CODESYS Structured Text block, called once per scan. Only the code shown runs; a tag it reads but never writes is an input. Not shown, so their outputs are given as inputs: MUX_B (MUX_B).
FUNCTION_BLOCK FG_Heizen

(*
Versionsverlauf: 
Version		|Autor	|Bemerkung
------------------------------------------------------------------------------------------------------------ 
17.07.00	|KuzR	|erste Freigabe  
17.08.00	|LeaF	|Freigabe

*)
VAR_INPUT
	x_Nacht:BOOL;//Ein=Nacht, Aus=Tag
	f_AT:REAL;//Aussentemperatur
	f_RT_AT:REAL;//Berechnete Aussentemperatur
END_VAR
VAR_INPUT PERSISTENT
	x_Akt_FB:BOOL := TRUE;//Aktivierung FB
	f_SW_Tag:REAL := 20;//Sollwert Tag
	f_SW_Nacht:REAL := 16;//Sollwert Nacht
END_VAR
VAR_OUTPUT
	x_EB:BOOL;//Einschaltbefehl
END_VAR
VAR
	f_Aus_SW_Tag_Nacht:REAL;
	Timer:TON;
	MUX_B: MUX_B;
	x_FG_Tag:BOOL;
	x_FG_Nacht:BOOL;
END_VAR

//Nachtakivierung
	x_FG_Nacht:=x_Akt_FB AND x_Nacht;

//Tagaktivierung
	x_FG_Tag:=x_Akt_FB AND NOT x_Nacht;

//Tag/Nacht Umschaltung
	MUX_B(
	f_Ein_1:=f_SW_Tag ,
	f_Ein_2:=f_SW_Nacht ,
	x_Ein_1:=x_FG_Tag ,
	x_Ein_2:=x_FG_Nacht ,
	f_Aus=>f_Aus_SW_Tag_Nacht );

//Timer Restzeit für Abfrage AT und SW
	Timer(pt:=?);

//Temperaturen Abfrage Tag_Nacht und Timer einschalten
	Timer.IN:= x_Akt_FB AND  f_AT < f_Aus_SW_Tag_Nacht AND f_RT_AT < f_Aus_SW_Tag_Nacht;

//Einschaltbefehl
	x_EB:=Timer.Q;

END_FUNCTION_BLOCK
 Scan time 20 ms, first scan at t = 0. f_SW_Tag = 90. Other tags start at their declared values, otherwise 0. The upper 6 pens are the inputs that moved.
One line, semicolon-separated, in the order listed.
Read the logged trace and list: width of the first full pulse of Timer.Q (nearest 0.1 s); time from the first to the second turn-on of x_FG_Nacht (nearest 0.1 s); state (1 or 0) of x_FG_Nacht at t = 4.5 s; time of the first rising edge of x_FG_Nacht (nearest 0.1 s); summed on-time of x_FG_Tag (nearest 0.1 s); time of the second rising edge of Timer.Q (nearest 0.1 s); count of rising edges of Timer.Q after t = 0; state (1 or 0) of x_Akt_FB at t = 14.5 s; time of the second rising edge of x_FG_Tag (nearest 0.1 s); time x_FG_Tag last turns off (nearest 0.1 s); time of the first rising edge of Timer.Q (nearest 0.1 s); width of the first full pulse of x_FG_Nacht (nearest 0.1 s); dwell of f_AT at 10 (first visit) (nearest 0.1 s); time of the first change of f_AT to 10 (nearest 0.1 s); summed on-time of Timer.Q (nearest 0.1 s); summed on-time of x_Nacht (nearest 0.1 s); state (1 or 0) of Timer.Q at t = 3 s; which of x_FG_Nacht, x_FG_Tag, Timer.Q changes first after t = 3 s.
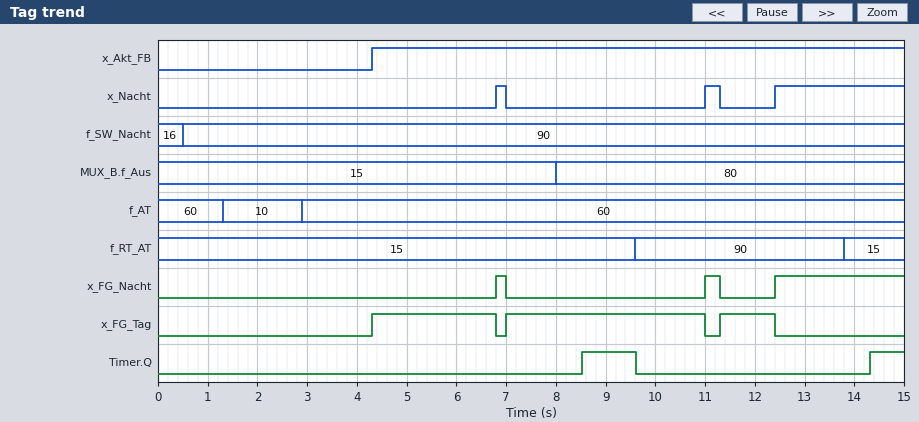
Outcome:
1.1 s; 4.2 s; 0; 6.8 s; 7.6 s; 14.3 s; 2; 1; 7.0 s; 12.4 s; 8.5 s; 0.2 s; 1.6 s; 1.3 s; 1.8 s; 3.1 s; 0; x_FG_Tag
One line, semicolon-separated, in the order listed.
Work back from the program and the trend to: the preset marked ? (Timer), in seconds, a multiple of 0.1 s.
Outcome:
0.5 s
